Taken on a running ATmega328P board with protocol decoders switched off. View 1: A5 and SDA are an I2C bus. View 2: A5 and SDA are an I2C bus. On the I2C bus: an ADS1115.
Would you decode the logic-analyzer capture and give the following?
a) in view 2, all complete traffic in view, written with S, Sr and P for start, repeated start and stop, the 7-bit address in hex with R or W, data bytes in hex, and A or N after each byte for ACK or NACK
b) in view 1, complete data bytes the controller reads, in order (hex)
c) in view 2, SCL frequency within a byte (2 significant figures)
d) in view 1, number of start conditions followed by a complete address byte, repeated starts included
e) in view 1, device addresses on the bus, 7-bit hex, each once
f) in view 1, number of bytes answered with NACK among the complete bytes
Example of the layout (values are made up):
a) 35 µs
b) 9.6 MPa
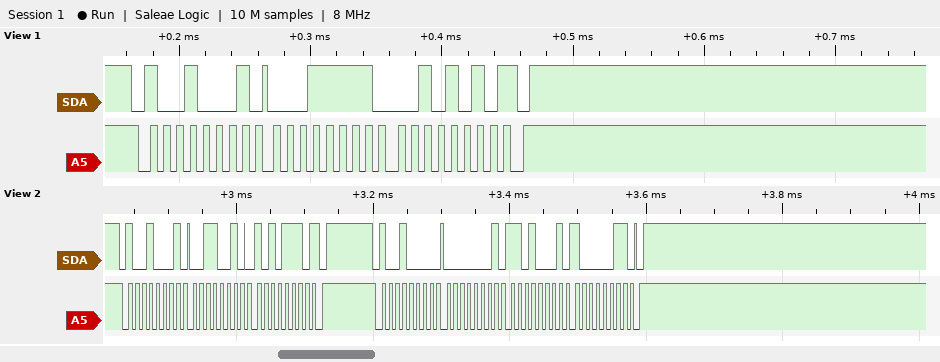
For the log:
a) S 48R A 32 A AE N P S 48W A 01 A D1 A 83 A P
b) 1F 2A
c) 100 kHz
d) 1
e) 0x48
f) 1
